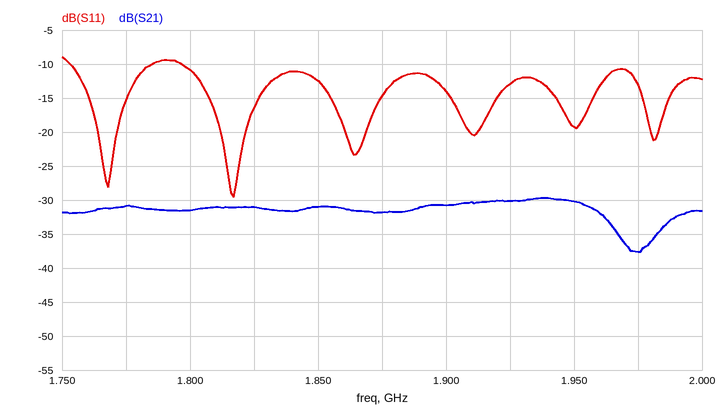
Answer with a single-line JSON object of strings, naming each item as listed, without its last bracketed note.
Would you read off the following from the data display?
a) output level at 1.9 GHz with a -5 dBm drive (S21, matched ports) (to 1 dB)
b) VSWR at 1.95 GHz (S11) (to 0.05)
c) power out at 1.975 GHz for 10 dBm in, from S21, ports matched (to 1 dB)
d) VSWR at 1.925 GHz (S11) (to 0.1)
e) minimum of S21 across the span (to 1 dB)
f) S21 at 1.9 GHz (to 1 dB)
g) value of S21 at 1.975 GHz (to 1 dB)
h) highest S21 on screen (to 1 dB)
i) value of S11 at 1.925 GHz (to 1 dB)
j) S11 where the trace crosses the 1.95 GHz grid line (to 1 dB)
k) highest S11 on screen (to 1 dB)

{"output level at 1.9 GHz with a -5 dBm drive (S21, matched ports)": "-36 dBm", "VSWR at 1.95 GHz (S11)": "1.25", "power out at 1.975 GHz for 10 dBm in, from S21, ports matched": "-28 dBm", "VSWR at 1.925 GHz (S11)": "1.6", "minimum of S21 across the span": "-38 dB", "S21 at 1.9 GHz": "-31 dB", "value of S21 at 1.975 GHz": "-38 dB", "highest S21 on screen": "-30 dB", "value of S11 at 1.925 GHz": "-13 dB", "S11 where the trace crosses the 1.95 GHz grid line": "-19 dB", "highest S11 on screen": "-9 dB"}
